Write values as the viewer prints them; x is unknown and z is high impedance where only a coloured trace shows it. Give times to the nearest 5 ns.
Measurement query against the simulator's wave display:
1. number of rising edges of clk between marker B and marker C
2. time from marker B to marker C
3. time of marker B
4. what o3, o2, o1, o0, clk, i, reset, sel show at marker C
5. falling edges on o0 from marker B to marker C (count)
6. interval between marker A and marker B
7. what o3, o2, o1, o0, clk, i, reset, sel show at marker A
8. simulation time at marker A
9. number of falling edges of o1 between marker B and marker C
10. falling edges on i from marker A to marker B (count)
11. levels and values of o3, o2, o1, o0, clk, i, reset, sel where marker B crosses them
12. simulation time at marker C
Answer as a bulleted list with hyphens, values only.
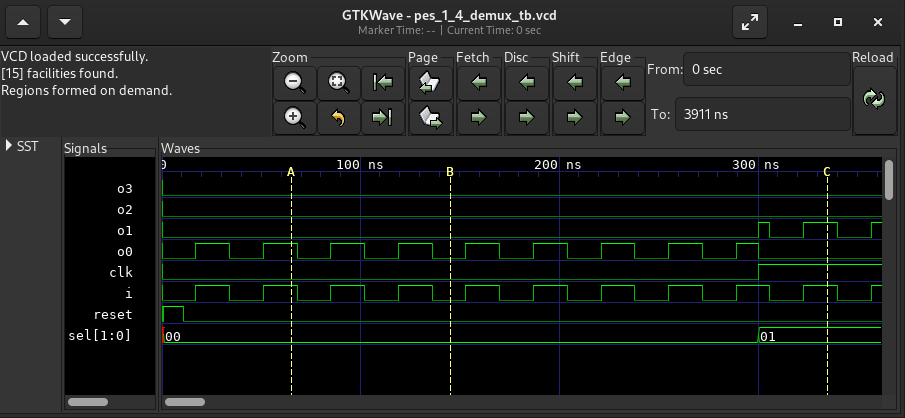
- 1
- 190 ns
- 145 ns
- o3=0, o2=0, o1=1, o0=0, clk=1, i=1, reset=0, sel=01
- 5
- 80 ns
- o3=0, o2=0, o1=0, o0=1, clk=0, i=1, reset=0, sel=00
- 65 ns
- 1
- 3
- o3=0, o2=0, o1=0, o0=0, clk=0, i=0, reset=0, sel=00
- 335 ns
